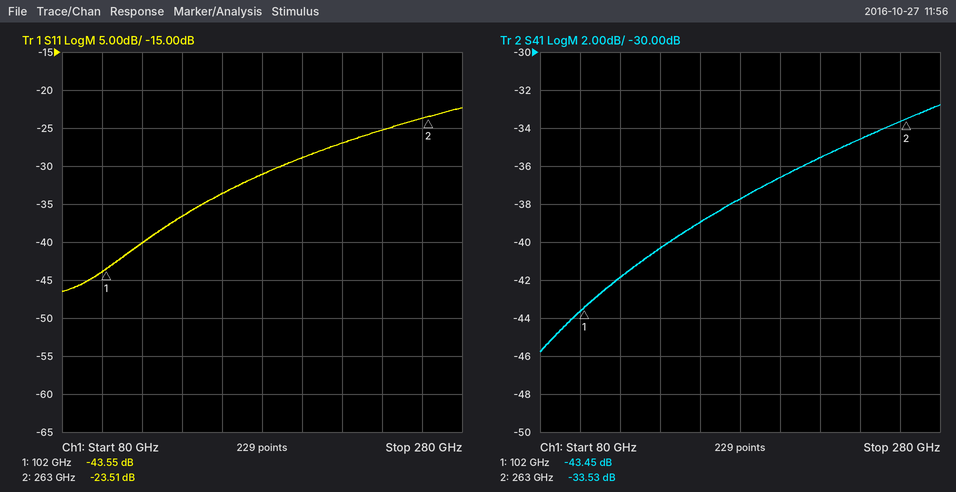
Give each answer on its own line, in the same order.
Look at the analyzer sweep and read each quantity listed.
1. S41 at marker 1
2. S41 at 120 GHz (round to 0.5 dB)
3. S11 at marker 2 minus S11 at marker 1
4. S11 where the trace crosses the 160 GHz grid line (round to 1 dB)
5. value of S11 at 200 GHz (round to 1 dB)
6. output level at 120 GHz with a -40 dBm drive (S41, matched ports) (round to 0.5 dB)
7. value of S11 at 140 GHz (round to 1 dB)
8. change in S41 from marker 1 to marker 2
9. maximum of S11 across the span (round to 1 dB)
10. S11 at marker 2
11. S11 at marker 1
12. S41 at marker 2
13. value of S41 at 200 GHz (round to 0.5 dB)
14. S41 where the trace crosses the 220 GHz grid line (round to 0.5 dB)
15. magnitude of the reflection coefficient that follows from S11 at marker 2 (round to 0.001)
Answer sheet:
-43.45 dB
-42.0 dB
20.04 dB
-34 dB
-29 dB
-82.0 dBm
-37 dB
9.92 dB
-22 dB
-23.51 dB
-43.55 dB
-33.53 dB
-36.5 dB
-35.5 dB
0.067
